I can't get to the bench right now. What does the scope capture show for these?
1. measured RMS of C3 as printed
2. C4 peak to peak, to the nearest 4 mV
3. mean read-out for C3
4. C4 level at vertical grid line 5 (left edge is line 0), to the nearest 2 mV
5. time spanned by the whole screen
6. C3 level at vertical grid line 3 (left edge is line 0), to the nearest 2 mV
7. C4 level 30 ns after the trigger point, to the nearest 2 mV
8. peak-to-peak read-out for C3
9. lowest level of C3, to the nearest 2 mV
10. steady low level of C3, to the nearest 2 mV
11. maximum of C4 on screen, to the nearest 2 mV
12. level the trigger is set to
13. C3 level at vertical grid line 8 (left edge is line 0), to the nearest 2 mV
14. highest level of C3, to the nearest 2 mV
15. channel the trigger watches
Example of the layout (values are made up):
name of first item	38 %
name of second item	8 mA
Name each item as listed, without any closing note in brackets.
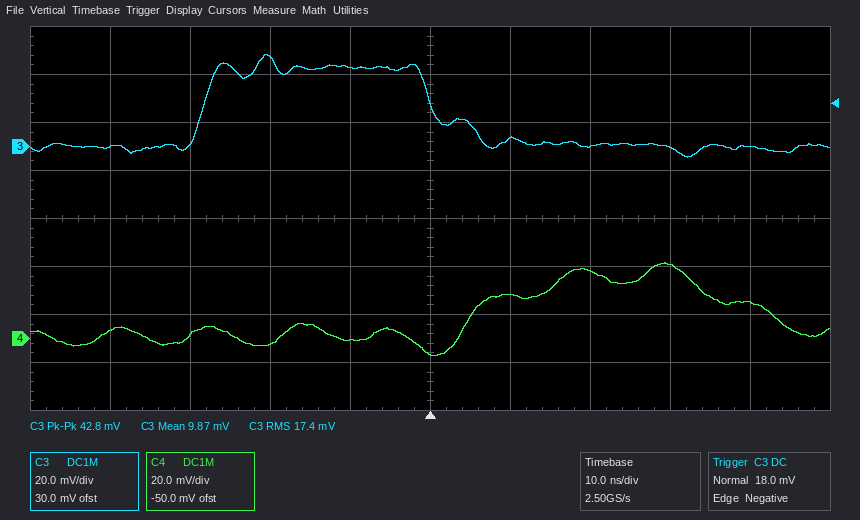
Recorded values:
measured RMS of C3 as printed	17.4 mV
C4 peak to peak, to the nearest 4 mV	40 mV
mean read-out for C3	9.87 mV
C4 level at vertical grid line 5 (left edge is line 0), to the nearest 2 mV	-6 mV
time spanned by the whole screen	100 ns
C3 level at vertical grid line 3 (left edge is line 0), to the nearest 2 mV	36 mV
C4 level 30 ns after the trigger point, to the nearest 2 mV	30 mV
peak-to-peak read-out for C3	42.8 mV
lowest level of C3, to the nearest 2 mV	-4 mV
steady low level of C3, to the nearest 2 mV	0 mV
maximum of C4 on screen, to the nearest 2 mV	32 mV
level the trigger is set to	18.0 mV
C3 level at vertical grid line 8 (left edge is line 0), to the nearest 2 mV	0 mV
highest level of C3, to the nearest 2 mV	38 mV
channel the trigger watches	C3
